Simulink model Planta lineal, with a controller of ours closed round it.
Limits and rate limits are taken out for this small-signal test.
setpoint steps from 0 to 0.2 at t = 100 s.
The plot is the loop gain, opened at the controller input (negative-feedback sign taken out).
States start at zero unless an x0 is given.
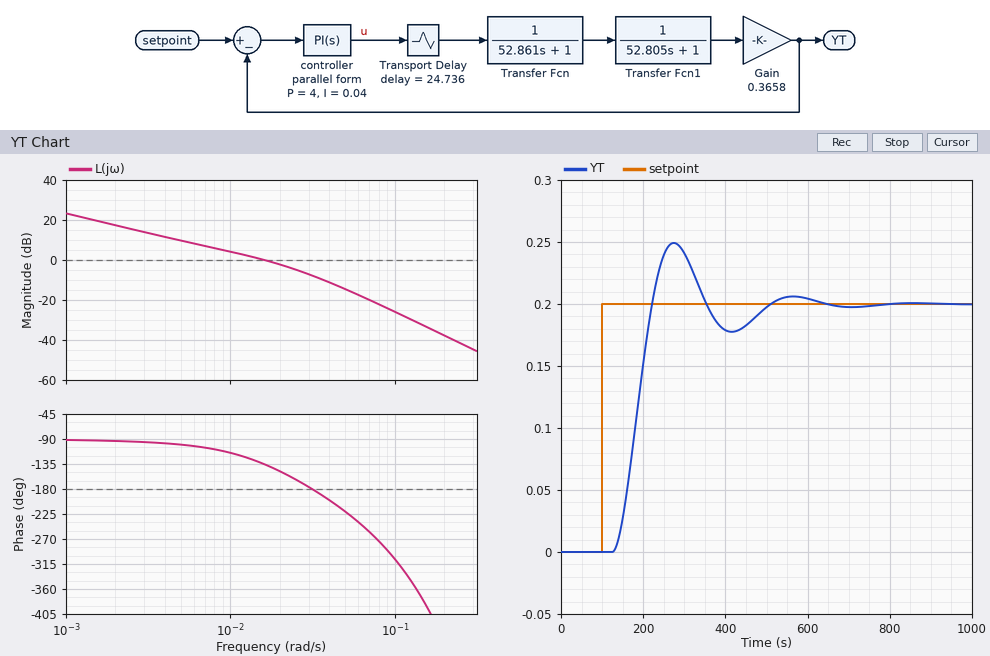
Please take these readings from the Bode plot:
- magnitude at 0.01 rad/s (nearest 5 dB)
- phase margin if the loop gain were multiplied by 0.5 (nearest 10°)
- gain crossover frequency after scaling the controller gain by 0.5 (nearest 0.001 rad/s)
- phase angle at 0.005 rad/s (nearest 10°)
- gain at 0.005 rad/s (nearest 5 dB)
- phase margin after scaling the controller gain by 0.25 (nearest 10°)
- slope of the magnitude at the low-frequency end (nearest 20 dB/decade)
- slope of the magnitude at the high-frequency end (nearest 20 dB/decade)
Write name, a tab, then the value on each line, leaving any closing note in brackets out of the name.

magnitude at 0.01 rad/s	5 dB
phase margin if the loop gain were multiplied by 0.5	70°
gain crossover frequency after scaling the controller gain by 0.5	0.008 rad/s
phase angle at 0.005 rad/s	-100°
gain at 0.005 rad/s	10 dB
phase margin after scaling the controller gain by 0.25	80°
slope of the magnitude at the low-frequency end	-20 dB/decade
slope of the magnitude at the high-frequency end	-40 dB/decade
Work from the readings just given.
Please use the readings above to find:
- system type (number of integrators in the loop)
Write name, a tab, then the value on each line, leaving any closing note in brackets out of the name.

system type	1
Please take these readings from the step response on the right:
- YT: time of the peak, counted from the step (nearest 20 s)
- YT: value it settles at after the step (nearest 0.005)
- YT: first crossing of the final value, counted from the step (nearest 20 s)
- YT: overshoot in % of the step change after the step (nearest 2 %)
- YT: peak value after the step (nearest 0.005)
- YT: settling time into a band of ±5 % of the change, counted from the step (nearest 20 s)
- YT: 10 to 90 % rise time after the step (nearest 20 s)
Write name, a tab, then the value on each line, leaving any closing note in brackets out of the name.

YT: time of the peak, counted from the step	180 s
YT: value it settles at after the step	0.200
YT: first crossing of the final value, counted from the step	120 s
YT: overshoot in % of the step change after the step	24 %
YT: peak value after the step	0.250
YT: settling time into a band of ±5 % of the change, counted from the step	380 s
YT: 10 to 90 % rise time after the step	60 s
